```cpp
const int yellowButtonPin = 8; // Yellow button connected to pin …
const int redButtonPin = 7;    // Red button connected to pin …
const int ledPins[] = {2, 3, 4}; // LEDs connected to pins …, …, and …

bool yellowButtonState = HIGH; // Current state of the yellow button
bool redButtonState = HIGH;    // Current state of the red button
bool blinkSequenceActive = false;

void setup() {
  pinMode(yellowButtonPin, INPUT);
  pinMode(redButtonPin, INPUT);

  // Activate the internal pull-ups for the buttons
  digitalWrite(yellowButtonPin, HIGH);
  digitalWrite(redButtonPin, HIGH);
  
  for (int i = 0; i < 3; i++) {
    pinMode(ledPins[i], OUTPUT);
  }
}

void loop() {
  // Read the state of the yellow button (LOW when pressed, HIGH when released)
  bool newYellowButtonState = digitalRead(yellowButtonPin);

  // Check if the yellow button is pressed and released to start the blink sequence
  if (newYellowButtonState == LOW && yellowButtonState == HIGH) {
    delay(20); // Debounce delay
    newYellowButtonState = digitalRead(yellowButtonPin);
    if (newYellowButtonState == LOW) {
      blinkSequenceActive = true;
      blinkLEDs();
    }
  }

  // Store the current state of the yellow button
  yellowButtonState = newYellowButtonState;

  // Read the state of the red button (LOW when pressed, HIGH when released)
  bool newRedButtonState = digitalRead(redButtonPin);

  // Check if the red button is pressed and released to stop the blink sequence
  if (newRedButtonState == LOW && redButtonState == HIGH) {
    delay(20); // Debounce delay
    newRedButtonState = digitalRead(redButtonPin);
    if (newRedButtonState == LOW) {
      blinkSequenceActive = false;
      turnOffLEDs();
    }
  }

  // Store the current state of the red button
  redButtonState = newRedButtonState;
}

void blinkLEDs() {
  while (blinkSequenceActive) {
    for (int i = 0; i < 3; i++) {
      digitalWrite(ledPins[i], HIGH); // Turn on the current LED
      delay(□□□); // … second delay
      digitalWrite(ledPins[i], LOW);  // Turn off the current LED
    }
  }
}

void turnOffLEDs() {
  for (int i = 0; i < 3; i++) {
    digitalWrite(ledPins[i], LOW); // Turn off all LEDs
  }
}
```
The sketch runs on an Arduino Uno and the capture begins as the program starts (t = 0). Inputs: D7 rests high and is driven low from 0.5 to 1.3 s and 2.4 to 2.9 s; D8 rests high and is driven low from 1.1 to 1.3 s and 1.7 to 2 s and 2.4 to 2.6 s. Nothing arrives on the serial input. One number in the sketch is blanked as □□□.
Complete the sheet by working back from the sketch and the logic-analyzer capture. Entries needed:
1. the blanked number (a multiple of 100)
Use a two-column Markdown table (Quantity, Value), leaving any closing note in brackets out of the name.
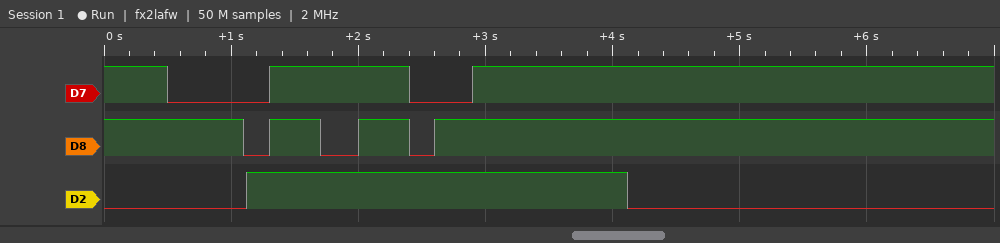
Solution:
| Quantity | Value |
|---|---|
| the blanked number | 3000 |
